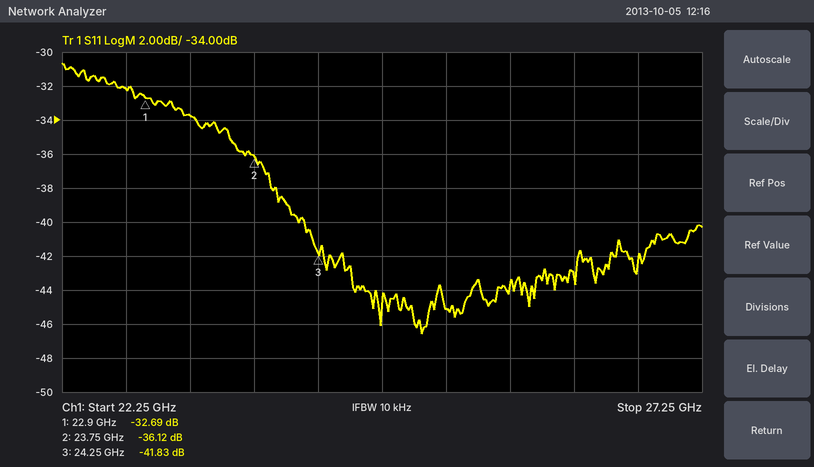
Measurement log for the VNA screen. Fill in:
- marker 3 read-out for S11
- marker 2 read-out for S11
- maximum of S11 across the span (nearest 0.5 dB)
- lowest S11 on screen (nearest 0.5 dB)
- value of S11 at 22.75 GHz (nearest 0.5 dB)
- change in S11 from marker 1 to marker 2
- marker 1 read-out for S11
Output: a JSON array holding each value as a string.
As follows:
["-41.83 dB", "-36.12 dB", "-30.5 dB", "-46.5 dB", "-32.0 dB", "-3.43 dB", "-32.69 dB"]
